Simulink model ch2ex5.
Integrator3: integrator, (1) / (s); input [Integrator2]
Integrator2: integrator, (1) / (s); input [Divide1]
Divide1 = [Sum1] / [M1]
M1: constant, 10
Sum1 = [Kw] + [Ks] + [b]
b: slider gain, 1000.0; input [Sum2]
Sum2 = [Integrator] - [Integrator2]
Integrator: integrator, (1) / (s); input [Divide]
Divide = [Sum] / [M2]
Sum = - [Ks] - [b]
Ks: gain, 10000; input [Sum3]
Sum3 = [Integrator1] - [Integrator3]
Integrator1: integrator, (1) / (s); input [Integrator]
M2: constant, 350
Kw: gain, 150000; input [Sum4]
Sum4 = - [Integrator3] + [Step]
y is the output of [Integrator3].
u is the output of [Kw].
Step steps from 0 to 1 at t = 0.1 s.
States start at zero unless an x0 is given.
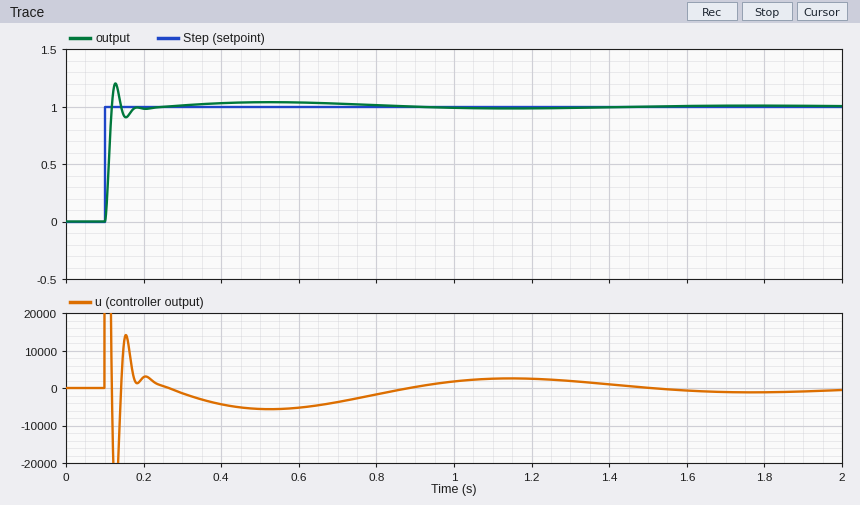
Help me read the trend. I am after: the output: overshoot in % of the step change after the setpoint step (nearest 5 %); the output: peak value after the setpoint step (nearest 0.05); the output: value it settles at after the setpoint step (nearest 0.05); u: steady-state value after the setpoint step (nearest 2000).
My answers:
20 %
1.20
1.00
0
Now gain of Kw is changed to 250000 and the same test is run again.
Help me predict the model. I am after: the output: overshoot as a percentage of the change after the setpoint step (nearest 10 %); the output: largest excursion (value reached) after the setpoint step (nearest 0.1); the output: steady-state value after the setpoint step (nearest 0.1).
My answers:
30 %
1.3
1.0
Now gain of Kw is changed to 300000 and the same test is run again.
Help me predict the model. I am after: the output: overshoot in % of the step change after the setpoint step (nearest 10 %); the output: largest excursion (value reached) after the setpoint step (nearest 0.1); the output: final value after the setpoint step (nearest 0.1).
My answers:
40 %
1.4
1.0
